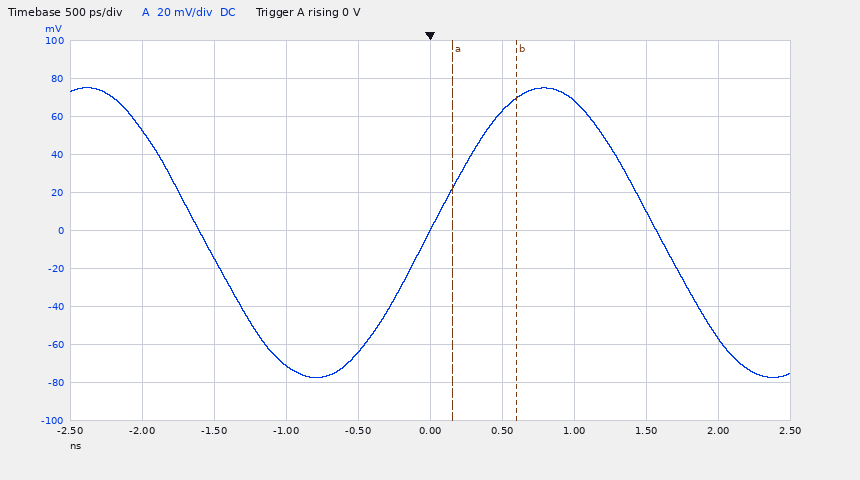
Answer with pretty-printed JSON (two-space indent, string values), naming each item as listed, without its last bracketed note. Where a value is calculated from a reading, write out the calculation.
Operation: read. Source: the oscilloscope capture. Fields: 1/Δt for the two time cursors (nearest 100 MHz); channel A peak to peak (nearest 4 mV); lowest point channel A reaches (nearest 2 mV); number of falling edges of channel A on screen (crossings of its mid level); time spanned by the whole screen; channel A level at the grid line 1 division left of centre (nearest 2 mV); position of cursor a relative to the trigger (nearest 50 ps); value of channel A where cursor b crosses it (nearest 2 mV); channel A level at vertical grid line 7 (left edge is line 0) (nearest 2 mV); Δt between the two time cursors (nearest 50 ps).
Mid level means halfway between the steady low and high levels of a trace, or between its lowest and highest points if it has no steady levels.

{
  "1/Δt for the two time cursors": "1 / 450 ps ≈ 2.2 GHz",
  "channel A peak to peak": "152 mV",
  "lowest point channel A reaches": "-78 mV",
  "number of falling edges of channel A on screen": "2",
  "time spanned by the whole screen": "5 ns",
  "channel A level at the grid line 1 division left of centre": "-64 mV",
  "position of cursor a relative to the trigger": "+150 ps",
  "value of channel A where cursor b crosses it": "70 mV",
  "channel A level at vertical grid line 7 (left edge is line 0)": "68 mV",
  "Δt between the two time cursors": "450 ps"
}
